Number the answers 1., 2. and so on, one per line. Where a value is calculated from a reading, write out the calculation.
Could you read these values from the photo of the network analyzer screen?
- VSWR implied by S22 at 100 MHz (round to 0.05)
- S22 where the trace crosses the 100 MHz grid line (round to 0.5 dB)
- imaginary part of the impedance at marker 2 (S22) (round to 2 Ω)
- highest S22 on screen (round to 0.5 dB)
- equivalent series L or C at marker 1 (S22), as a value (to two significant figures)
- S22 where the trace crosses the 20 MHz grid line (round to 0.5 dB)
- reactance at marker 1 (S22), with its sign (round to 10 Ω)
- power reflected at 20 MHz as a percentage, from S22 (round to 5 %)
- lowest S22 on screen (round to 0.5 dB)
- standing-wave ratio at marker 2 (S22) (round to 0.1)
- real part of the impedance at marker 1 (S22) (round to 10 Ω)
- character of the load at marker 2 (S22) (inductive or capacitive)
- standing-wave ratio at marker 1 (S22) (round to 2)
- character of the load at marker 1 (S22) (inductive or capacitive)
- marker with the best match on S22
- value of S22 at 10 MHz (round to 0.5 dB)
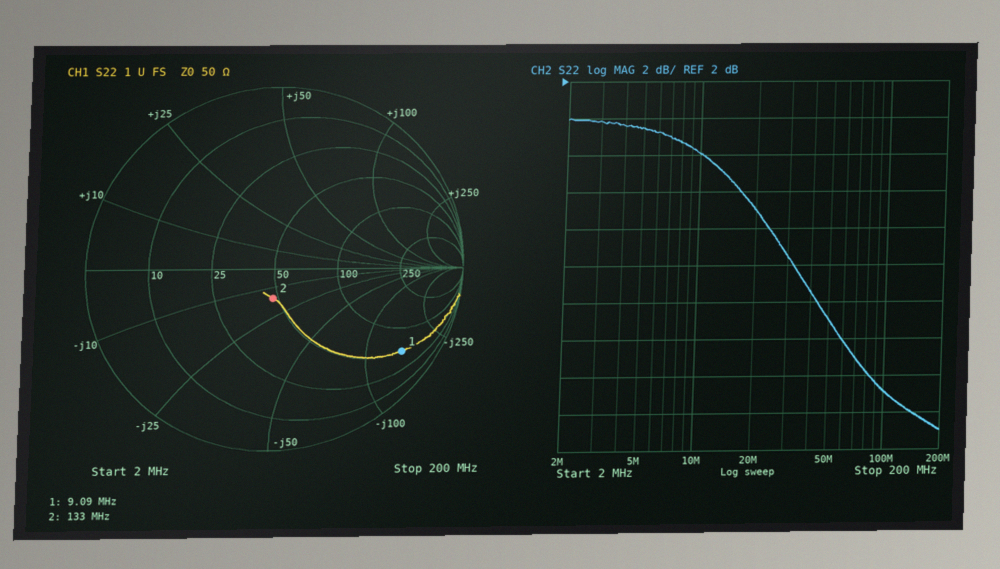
1. |Γ| = 10^(-15/20) = 0.1778; VSWR = (1 + 0.1778)/(1 − 0.1778) ≈ 1.43, so 1.45 to the nearest 0.05
2. -15.0 dB
3. -16 Ω
4. 0.0 dB
5. C = 1/(2π × 9.09 MHz × 150 Ω) ≈ 117 pF, so 120 pF to two significant figures
6. -5.0 dB
7. -150 Ω
8. 10^(-5/10) ≈ 31.6 %, so 30 % to the nearest 5 %
9. -17.0 dB
10. 1.4
11. 50 Ω
12. capacitive
13. 10
14. capacitive
15. marker 2
16. -2.0 dB
